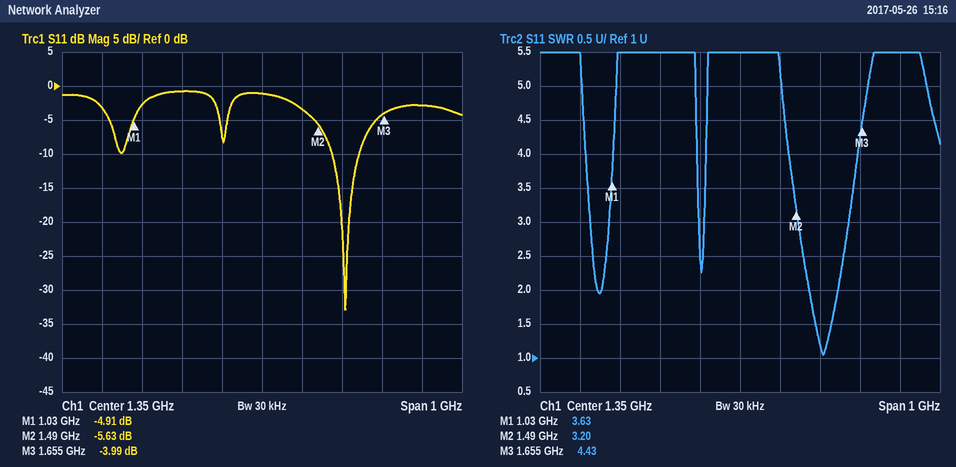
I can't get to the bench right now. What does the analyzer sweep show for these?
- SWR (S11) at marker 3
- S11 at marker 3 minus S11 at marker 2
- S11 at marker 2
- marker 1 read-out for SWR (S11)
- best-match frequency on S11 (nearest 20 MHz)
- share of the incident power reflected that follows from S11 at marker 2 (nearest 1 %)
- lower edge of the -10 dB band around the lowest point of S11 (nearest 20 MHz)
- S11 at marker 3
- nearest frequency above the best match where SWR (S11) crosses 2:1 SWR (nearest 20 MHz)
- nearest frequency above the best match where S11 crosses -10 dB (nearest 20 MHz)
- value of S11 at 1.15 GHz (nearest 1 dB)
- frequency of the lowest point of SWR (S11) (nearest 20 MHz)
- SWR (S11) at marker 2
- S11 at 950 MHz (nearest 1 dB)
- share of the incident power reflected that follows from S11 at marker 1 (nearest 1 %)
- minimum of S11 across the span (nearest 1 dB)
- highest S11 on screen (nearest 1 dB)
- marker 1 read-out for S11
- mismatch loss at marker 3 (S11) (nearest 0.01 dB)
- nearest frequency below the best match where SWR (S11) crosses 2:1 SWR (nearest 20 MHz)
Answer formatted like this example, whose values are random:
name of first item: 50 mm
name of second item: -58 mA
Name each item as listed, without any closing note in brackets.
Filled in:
SWR (S11) at marker 3: 4.43
S11 at marker 3 minus S11 at marker 2: 1.64 dB
S11 at marker 2: -5.63 dB
marker 1 read-out for SWR: 3.63
best-match frequency on S11: 1.56 GHz
share of the incident power reflected that follows from S11 at marker 2: 27 %
lower edge of the -10 dB band around the lowest point of S11: 1.52 GHz
S11 at marker 3: -3.99 dB
nearest frequency above the best match where SWR (S11) crosses 2:1 SWR: 1.60 GHz
nearest frequency above the best match where S11 crosses -10 dB: 1.60 GHz
value of S11 at 1.15 GHz: -1 dB
frequency of the lowest point of SWR (S11): 1.56 GHz
SWR (S11) at marker 2: 3.20
S11 at 950 MHz: -3 dB
share of the incident power reflected that follows from S11 at marker 1: 32 %
minimum of S11 across the span: -33 dB
highest S11 on screen: -1 dB
marker 1 read-out for S11: -4.91 dB
mismatch loss at marker 3 (S11): 2.21 dB
nearest frequency below the best match where SWR (S11) crosses 2:1 SWR: 1.52 GHz
